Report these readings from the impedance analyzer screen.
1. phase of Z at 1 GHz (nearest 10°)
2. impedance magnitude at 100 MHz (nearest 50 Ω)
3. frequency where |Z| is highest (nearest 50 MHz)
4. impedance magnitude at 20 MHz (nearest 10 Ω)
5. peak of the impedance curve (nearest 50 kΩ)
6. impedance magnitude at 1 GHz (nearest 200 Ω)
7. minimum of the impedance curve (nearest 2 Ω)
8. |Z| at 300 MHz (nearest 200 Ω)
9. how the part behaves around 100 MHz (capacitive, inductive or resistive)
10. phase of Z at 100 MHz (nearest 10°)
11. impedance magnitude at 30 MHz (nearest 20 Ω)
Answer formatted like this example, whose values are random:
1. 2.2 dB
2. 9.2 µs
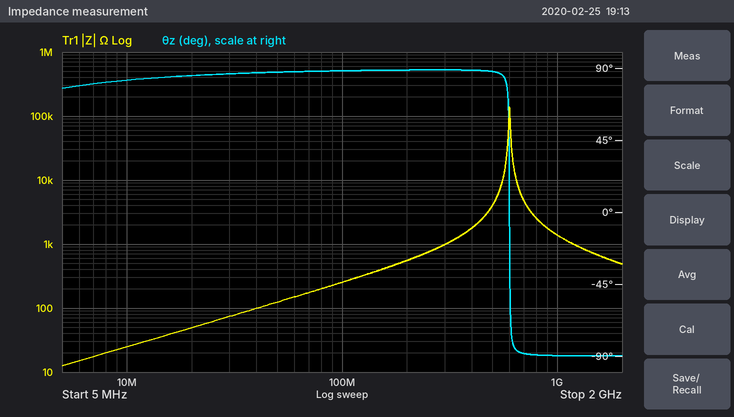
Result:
1. -90°
2. 250 Ω
3. 600 MHz
4. 50 Ω
5. 150 kΩ
6. 1.4 kΩ
7. 12 Ω
8. 1.0 kΩ
9. inductive
10. 90°
11. 80 Ω
